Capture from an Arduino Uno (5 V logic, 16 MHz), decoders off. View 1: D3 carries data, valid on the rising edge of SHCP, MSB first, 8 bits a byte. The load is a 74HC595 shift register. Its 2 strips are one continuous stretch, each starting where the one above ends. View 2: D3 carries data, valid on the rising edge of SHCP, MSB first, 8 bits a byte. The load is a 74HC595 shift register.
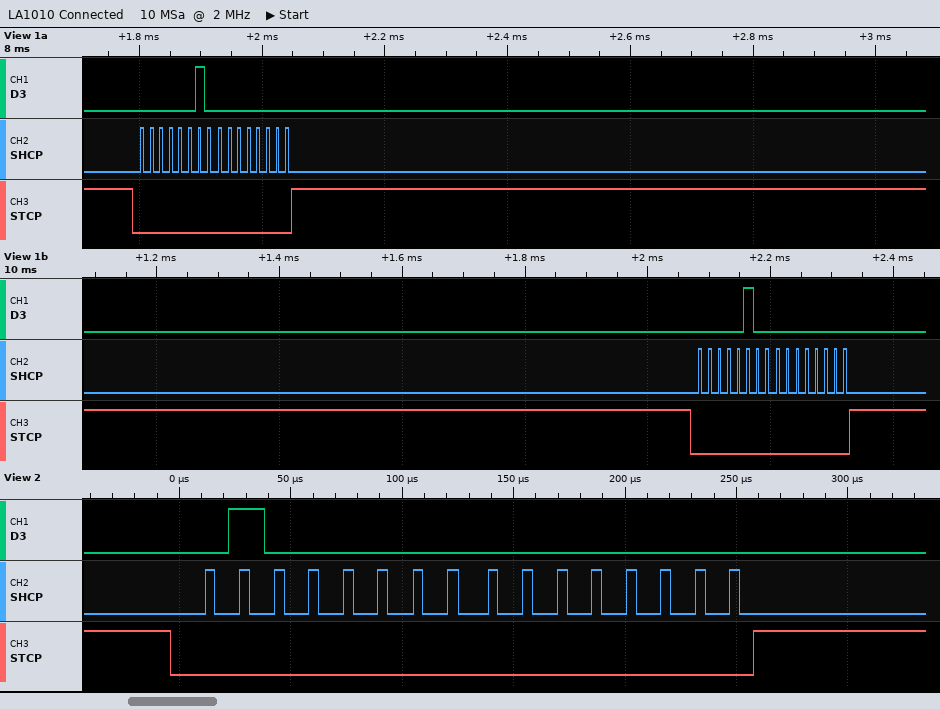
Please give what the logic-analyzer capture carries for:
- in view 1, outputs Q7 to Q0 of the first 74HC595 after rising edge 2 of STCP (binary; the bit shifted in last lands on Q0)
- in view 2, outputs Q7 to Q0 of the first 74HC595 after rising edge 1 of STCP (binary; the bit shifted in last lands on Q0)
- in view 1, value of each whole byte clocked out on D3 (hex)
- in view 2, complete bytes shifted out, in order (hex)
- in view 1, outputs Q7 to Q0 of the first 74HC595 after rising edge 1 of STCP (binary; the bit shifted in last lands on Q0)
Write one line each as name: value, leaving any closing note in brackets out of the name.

in view 1, outputs Q7 to Q0 of the first 74HC595 after rising edge 2 of STCP: 00000000
in view 2, outputs Q7 to Q0 of the first 74HC595 after rising edge 1 of STCP: 00000000
in view 1, value of each whole byte clocked out on D3: 0x02 0x00 0x04 0x00
in view 2, complete bytes shifted out, in order: 40 00
in view 1, outputs Q7 to Q0 of the first 74HC595 after rising edge 1 of STCP: 00000000
